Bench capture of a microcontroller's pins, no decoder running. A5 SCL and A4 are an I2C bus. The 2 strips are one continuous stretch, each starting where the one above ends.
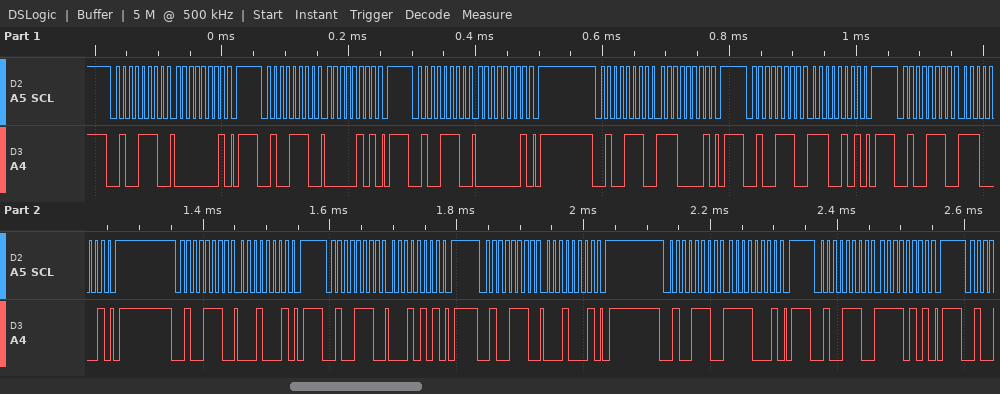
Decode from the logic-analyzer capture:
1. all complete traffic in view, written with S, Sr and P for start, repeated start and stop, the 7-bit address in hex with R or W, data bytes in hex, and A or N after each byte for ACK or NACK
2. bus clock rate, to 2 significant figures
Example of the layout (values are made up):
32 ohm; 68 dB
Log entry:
S 27W A 01 A P S 27W A 05 A P S 27W A 01 A P S 27W A E1 A P S 27W A E5 A P S 27W A E1 A P S 27W A 11 A P S 27W A 15 A P S 27W A 11 A P S 27W A F1 A P S 27W A F5 A P; 100 kHz
